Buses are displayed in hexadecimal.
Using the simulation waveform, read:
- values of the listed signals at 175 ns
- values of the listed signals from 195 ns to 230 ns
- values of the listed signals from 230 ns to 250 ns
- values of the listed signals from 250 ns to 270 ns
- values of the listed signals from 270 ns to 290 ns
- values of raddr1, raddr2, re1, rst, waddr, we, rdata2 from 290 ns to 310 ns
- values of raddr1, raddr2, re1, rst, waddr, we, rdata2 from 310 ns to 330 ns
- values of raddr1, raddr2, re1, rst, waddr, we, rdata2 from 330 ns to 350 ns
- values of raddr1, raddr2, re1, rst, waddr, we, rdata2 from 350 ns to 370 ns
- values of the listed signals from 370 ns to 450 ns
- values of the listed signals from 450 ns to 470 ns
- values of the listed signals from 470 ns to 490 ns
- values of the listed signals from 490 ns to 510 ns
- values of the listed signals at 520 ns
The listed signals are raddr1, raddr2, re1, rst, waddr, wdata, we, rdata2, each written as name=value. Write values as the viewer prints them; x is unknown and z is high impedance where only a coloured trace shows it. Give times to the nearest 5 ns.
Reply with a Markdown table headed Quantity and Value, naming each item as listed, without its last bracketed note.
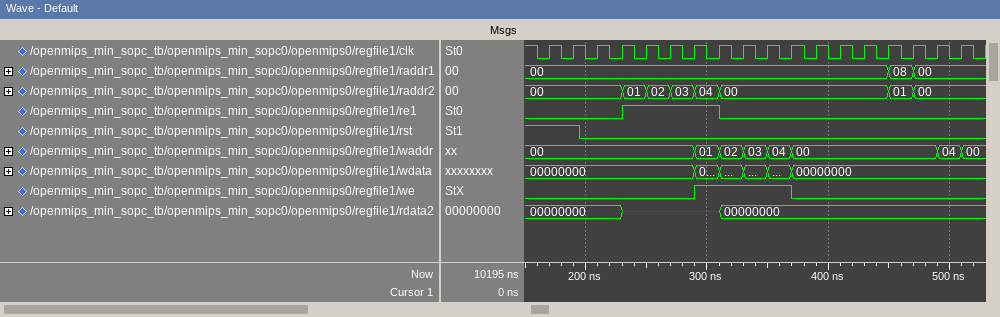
| Quantity | Value |
|---|---|
| values of the listed signals at 175 ns | raddr1=00, raddr2=00, re1=0, rst=1, waddr=00, wdata=00000000, we=0, rdata2=00000000 |
| values of the listed signals from 195 ns to 230 ns | raddr1=00, raddr2=00, re1=0, rst=0, waddr=00, wdata=00000000, we=0, rdata2=00000000 |
| values of the listed signals from 230 ns to 250 ns | raddr1=00, raddr2=01, re1=1, rst=0, waddr=00, wdata=00000000, we=0, rdata2=x |
| values of the listed signals from 250 ns to 270 ns | raddr1=00, raddr2=02, re1=1, rst=0, waddr=00, wdata=00000000, we=0, rdata2=x |
| values of the listed signals from 270 ns to 290 ns | raddr1=00, raddr2=03, re1=1, rst=0, waddr=00, wdata=00000000, we=0, rdata2=x |
| values of raddr1, raddr2, re1, rst, waddr, we, rdata2 from 290 ns to 310 ns | raddr1=00, raddr2=04, re1=1, rst=0, waddr=01, we=1, rdata2=x |
| values of raddr1, raddr2, re1, rst, waddr, we, rdata2 from 310 ns to 330 ns | raddr1=00, raddr2=00, re1=0, rst=0, waddr=02, we=1, rdata2=00000000 |
| values of raddr1, raddr2, re1, rst, waddr, we, rdata2 from 330 ns to 350 ns | raddr1=00, raddr2=00, re1=0, rst=0, waddr=03, we=1, rdata2=00000000 |
| values of raddr1, raddr2, re1, rst, waddr, we, rdata2 from 350 ns to 370 ns | raddr1=00, raddr2=00, re1=0, rst=0, waddr=04, we=1, rdata2=00000000 |
| values of the listed signals from 370 ns to 450 ns | raddr1=00, raddr2=00, re1=0, rst=0, waddr=00, wdata=00000000, we=0, rdata2=00000000 |
| values of the listed signals from 450 ns to 470 ns | raddr1=08, raddr2=01, re1=0, rst=0, waddr=00, wdata=00000000, we=0, rdata2=00000000 |
| values of the listed signals from 470 ns to 490 ns | raddr1=00, raddr2=00, re1=0, rst=0, waddr=00, wdata=00000000, we=0, rdata2=00000000 |
| values of the listed signals from 490 ns to 510 ns | raddr1=00, raddr2=00, re1=0, rst=0, waddr=04, wdata=00000000, we=0, rdata2=00000000 |
| values of the listed signals at 520 ns | raddr1=00, raddr2=00, re1=0, rst=0, waddr=00, wdata=00000000, we=0, rdata2=00000000 |
